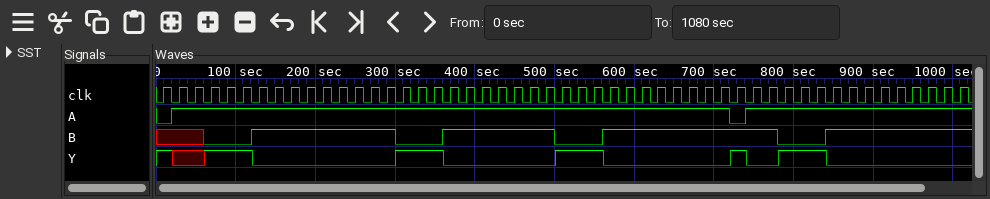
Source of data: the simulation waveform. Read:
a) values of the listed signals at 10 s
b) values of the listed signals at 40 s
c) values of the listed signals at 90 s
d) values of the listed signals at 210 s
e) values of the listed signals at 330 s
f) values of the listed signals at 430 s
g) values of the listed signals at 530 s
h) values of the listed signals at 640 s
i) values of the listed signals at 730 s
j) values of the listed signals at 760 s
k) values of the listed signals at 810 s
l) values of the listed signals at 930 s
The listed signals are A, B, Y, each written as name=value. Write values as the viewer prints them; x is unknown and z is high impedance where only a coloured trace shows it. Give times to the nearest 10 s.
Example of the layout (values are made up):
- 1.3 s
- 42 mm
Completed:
- A=0, B=x, Y=1
- A=1, B=x, Y=x
- A=1, B=0, Y=1
- A=1, B=1, Y=0
- A=1, B=0, Y=1
- A=1, B=1, Y=0
- A=1, B=0, Y=1
- A=1, B=1, Y=0
- A=0, B=1, Y=1
- A=1, B=1, Y=0
- A=1, B=0, Y=1
- A=1, B=1, Y=0
